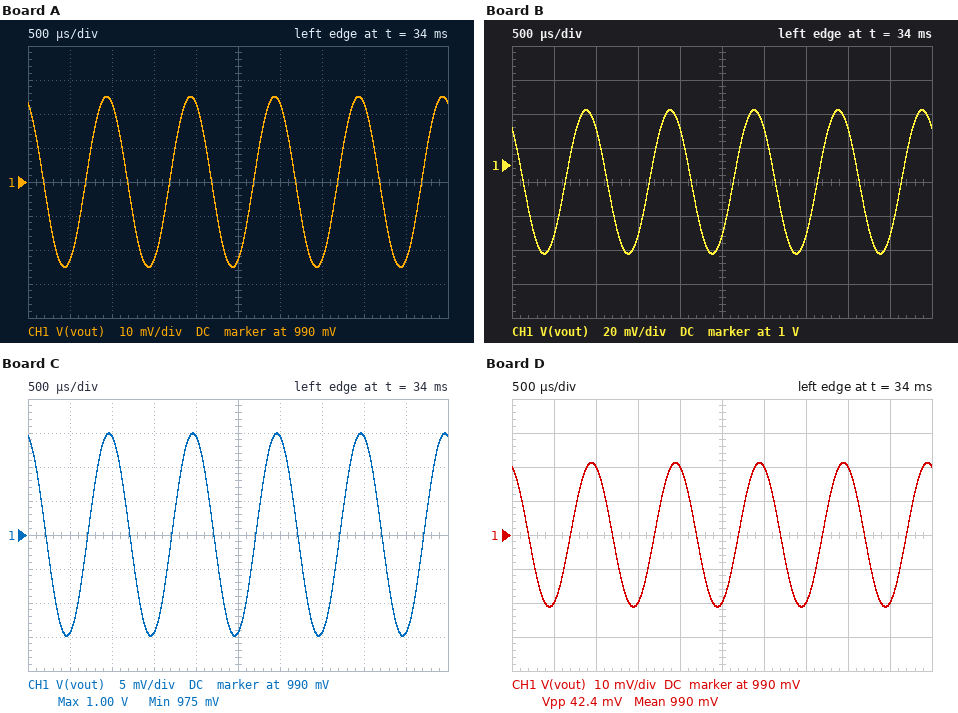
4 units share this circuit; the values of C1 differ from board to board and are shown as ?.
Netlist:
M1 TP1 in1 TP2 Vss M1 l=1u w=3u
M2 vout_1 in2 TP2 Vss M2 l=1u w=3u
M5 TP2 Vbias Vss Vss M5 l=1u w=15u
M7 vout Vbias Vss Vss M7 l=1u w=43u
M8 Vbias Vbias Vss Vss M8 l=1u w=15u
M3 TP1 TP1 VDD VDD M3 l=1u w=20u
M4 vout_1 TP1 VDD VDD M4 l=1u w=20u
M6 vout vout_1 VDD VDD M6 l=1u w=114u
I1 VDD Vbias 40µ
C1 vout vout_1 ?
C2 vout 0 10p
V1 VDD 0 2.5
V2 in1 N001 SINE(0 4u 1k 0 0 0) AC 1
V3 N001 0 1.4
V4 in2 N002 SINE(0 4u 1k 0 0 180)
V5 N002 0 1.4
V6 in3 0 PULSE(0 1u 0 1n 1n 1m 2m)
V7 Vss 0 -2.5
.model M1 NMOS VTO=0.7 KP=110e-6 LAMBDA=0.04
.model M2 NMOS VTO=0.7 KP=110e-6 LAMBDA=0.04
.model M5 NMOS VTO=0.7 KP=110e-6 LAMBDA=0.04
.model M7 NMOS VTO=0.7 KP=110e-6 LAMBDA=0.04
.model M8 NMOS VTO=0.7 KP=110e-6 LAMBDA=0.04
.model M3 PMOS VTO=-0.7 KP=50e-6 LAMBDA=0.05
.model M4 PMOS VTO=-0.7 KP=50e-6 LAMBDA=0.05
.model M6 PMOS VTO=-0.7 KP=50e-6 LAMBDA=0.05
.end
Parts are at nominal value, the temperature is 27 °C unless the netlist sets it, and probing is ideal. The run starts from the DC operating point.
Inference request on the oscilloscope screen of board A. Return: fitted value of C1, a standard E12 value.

5.6 pF
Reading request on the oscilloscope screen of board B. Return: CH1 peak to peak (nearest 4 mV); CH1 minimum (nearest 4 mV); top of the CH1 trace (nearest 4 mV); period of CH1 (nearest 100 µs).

84 mV
948 mV
1.032 V
1.0 ms
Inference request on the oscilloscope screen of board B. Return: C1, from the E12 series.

2.7 pF
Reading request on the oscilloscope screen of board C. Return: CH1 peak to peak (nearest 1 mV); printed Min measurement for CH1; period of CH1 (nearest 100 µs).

30 mV
975 mV
1.0 ms
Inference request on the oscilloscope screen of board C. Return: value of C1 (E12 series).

10 pF
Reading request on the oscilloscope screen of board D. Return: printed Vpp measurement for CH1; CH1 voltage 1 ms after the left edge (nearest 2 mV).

42.4 mV
1.010 V
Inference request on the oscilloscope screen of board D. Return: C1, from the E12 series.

6.8 pF
